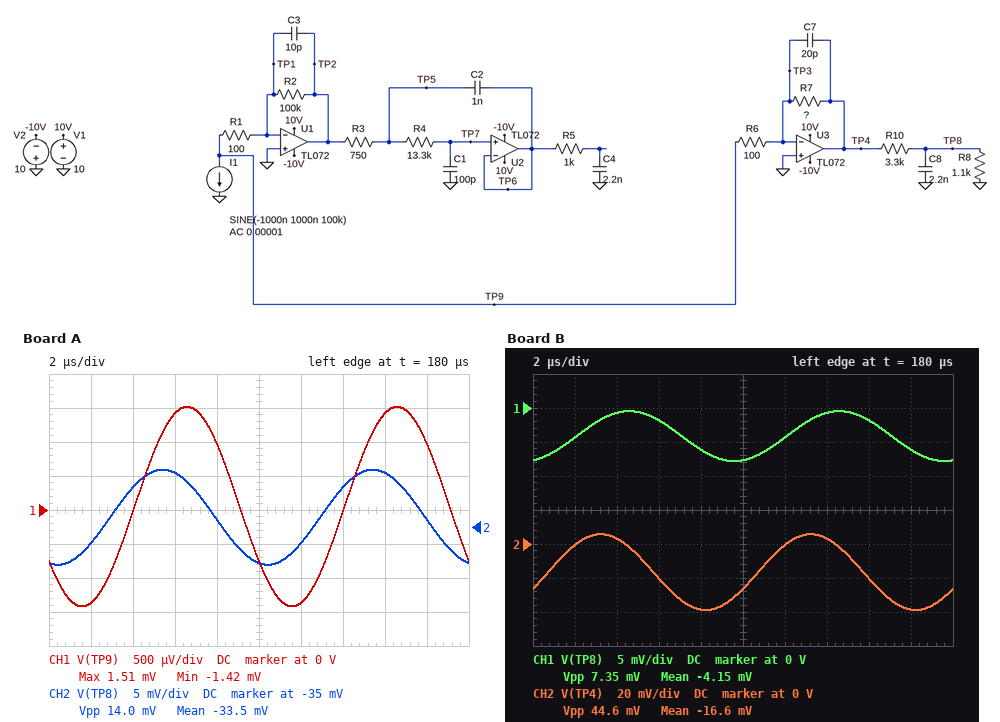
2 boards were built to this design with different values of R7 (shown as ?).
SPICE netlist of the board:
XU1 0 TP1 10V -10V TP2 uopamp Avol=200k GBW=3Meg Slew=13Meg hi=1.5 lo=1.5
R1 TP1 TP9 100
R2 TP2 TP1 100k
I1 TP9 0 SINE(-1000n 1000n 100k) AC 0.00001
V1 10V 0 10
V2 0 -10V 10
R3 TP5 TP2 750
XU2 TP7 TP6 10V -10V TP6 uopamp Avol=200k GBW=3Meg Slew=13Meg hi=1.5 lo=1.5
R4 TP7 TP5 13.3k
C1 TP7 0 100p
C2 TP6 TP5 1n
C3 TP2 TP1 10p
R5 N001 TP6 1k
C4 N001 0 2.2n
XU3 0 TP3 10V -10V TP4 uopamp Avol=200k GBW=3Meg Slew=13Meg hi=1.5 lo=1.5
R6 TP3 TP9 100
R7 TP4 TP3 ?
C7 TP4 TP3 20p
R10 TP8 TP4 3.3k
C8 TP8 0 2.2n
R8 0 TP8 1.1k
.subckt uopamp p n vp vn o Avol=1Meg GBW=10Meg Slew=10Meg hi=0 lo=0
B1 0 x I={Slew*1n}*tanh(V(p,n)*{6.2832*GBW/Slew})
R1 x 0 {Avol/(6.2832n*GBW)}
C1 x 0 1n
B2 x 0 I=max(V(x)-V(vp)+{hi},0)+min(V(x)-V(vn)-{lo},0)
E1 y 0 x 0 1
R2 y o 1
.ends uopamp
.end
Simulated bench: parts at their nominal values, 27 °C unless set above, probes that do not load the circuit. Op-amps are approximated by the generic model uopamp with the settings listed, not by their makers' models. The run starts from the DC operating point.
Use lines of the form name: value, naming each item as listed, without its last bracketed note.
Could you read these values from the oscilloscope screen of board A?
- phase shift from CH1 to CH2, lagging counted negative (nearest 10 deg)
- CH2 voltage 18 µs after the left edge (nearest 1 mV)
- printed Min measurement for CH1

phase shift from CH1 to CH2, lagging counted negative: 40 deg
CH2 voltage 18 µs after the left edge: -34 mV
printed Min measurement for CH1: -1.42 mV
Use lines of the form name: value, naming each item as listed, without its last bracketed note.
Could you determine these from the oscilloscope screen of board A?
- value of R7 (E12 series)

value of R7: 270 kΩ
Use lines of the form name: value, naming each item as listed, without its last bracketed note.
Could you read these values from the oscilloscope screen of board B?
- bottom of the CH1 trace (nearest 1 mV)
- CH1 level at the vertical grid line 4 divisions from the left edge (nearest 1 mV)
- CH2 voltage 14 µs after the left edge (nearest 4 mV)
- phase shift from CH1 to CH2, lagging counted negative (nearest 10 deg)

bottom of the CH1 trace: -8 mV
CH1 level at the vertical grid line 4 divisions from the left edge: -6 mV
CH2 voltage 14 µs after the left edge: 4 mV
phase shift from CH1 to CH2, lagging counted negative: 50 deg
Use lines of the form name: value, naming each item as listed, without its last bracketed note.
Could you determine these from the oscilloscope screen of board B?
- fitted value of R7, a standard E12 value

fitted value of R7, a standard E12 value: 33 kΩ
